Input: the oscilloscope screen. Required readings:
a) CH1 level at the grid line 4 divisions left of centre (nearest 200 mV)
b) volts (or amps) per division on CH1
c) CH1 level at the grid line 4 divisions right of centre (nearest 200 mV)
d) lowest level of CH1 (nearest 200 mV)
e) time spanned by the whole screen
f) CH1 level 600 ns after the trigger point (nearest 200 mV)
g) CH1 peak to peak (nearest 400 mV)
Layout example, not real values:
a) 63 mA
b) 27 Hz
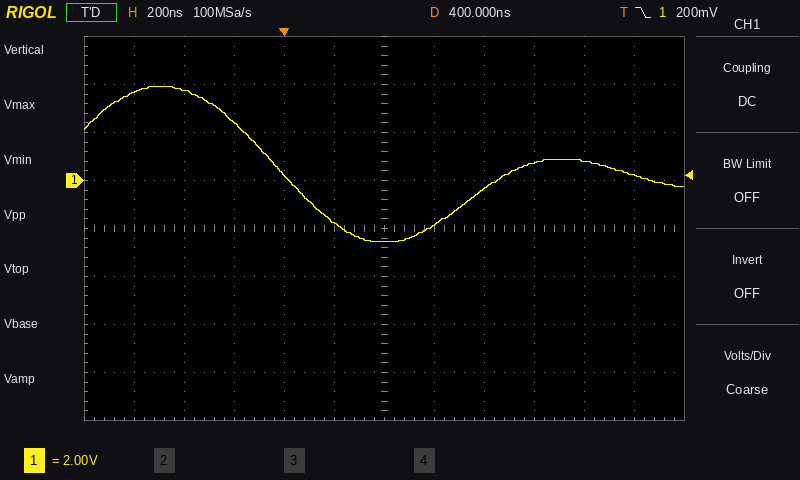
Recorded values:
a) 3.8 V
b) 2 V
c) 800 mV
d) -2.6 V
e) 2.4 µs
f) -1.8 V
g) 6.4 V
